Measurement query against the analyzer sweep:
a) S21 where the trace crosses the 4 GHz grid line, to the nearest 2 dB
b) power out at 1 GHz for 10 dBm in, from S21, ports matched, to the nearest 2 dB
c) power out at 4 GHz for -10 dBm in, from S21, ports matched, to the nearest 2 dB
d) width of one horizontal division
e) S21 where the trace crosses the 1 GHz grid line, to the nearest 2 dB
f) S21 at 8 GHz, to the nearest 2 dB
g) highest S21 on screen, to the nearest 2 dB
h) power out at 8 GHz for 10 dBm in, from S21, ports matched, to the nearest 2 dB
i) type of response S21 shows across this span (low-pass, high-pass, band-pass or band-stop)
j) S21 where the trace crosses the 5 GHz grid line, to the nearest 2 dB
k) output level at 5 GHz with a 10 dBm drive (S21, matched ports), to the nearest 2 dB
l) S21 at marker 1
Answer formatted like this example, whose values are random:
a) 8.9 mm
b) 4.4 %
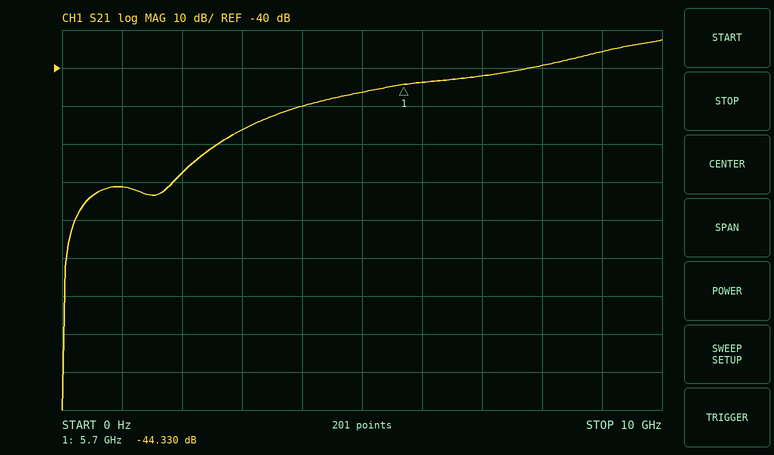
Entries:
a) -50 dB
b) -62 dBm
c) -60 dBm
d) 1 GHz
e) -72 dB
f) -40 dB
g) -32 dB
h) -30 dBm
i) high-pass
j) -46 dB
k) -36 dBm
l) -44.330 dB
